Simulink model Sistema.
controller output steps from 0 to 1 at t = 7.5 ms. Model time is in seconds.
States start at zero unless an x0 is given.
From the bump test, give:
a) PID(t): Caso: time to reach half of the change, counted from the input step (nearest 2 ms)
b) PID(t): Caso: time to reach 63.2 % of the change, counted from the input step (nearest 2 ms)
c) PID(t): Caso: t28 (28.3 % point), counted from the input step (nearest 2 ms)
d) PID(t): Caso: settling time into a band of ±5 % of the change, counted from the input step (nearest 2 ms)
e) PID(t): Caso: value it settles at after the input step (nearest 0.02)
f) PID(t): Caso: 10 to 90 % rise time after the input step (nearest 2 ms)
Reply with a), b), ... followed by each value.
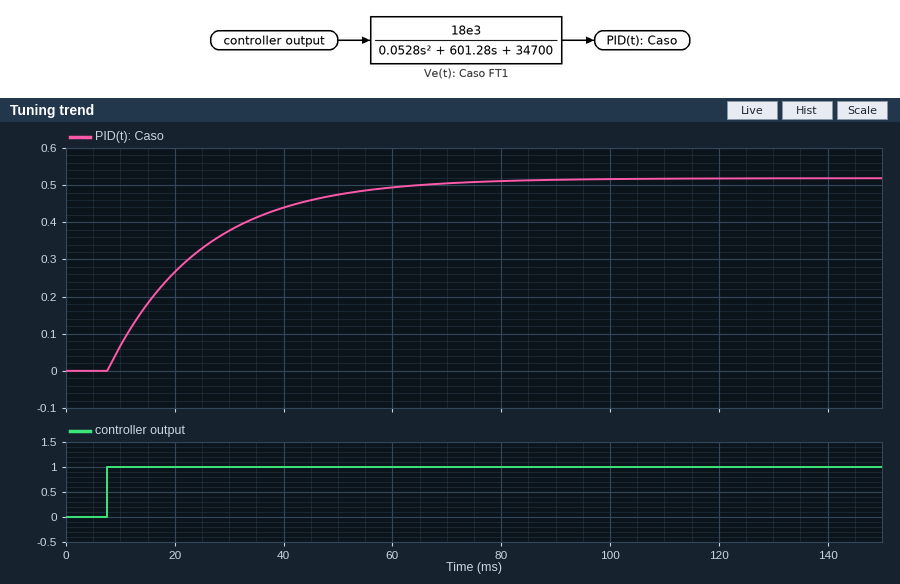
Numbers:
a) 12 ms
b) 18 ms
c) 6 ms
d) 52 ms
e) 0.52
f) 38 ms
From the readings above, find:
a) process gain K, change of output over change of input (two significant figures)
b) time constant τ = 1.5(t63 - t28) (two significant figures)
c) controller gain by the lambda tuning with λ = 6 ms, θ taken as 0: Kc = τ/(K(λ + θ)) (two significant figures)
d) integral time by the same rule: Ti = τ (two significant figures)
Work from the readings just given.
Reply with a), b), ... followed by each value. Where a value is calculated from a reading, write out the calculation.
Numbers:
a) (0.52 - 0) / 1 = 0.52
b) 1.5 × (18 - 6) = 18 ms
c) 18 / (0.52 × (6 + 0)) = 5.8
d) 18 ms
